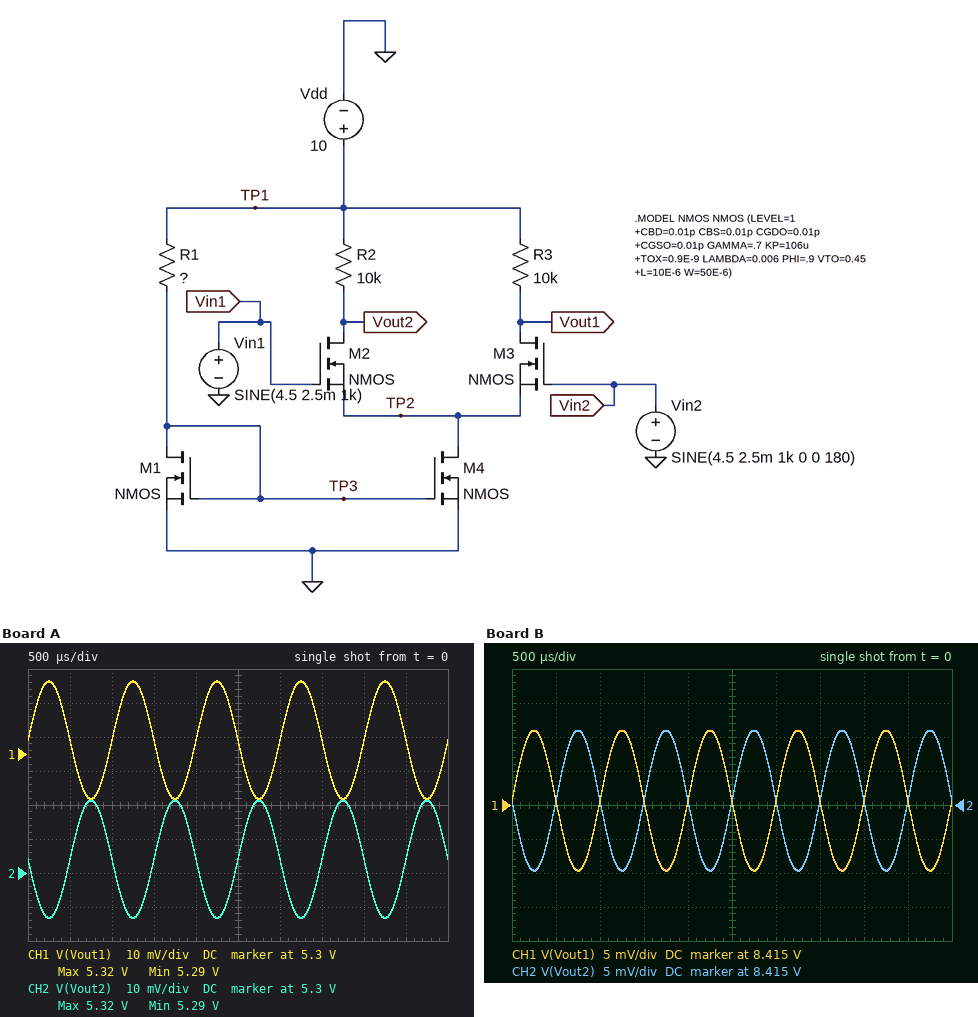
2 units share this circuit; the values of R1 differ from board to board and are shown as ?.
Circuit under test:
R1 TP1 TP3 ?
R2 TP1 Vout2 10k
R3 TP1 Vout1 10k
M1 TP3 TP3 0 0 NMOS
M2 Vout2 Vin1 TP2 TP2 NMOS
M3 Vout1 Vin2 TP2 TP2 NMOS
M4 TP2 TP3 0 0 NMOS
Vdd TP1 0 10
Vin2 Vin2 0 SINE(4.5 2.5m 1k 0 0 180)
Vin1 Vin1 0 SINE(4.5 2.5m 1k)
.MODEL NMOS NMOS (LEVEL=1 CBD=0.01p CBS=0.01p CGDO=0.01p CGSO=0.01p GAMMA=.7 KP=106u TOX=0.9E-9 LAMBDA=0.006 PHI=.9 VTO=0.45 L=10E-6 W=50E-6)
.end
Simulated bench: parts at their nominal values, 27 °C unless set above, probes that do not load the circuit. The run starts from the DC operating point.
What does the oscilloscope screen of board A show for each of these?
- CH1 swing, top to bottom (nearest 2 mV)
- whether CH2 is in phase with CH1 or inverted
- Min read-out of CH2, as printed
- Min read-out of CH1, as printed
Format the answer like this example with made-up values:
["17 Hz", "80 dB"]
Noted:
["34 mV", "inverted", "5.29 V", "5.29 V"]
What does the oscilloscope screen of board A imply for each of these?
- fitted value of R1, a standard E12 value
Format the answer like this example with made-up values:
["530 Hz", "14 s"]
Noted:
["8.2 kΩ"]
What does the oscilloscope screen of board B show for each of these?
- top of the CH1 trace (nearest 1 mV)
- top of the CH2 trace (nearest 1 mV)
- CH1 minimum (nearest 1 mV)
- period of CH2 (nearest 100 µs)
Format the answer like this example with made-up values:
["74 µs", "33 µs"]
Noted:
["8.426 V", "8.426 V", "8.405 V", "1.0 ms"]
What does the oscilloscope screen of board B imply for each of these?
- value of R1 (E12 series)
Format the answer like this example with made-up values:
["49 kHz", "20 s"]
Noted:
["27 kΩ"]
